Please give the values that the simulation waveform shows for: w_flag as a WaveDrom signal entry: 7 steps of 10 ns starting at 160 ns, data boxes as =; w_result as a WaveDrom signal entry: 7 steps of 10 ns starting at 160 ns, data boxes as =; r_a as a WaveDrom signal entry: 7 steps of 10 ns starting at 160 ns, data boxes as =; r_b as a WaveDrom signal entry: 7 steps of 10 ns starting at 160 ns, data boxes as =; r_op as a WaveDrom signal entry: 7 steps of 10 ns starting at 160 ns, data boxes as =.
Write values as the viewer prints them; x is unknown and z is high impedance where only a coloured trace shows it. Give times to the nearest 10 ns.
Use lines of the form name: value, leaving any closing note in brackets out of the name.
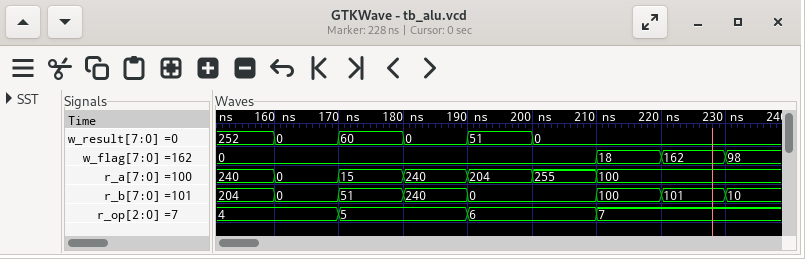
w_flag as a WaveDrom signal entry: 7 steps of 10 ns starting at 160 ns, data boxes as =: {name: 'w_flag', wave: '=....==', data: '0 18 162'}
w_result as a WaveDrom signal entry: 7 steps of 10 ns starting at 160 ns, data boxes as =: {name: 'w_result', wave: '=====..', data: '0 60 0 51 0'}
r_a as a WaveDrom signal entry: 7 steps of 10 ns starting at 160 ns, data boxes as =: {name: 'r_a', wave: '======.', data: '0 15 240 204 255 100'}
r_b as a WaveDrom signal entry: 7 steps of 10 ns starting at 160 ns, data boxes as =: {name: 'r_b', wave: '====.==', data: '0 51 240 0 100 101'}
r_op as a WaveDrom signal entry: 7 steps of 10 ns starting at 160 ns, data boxes as =: {name: 'r_op', wave: '==.=.=.', data: '4 5 6 7'}
